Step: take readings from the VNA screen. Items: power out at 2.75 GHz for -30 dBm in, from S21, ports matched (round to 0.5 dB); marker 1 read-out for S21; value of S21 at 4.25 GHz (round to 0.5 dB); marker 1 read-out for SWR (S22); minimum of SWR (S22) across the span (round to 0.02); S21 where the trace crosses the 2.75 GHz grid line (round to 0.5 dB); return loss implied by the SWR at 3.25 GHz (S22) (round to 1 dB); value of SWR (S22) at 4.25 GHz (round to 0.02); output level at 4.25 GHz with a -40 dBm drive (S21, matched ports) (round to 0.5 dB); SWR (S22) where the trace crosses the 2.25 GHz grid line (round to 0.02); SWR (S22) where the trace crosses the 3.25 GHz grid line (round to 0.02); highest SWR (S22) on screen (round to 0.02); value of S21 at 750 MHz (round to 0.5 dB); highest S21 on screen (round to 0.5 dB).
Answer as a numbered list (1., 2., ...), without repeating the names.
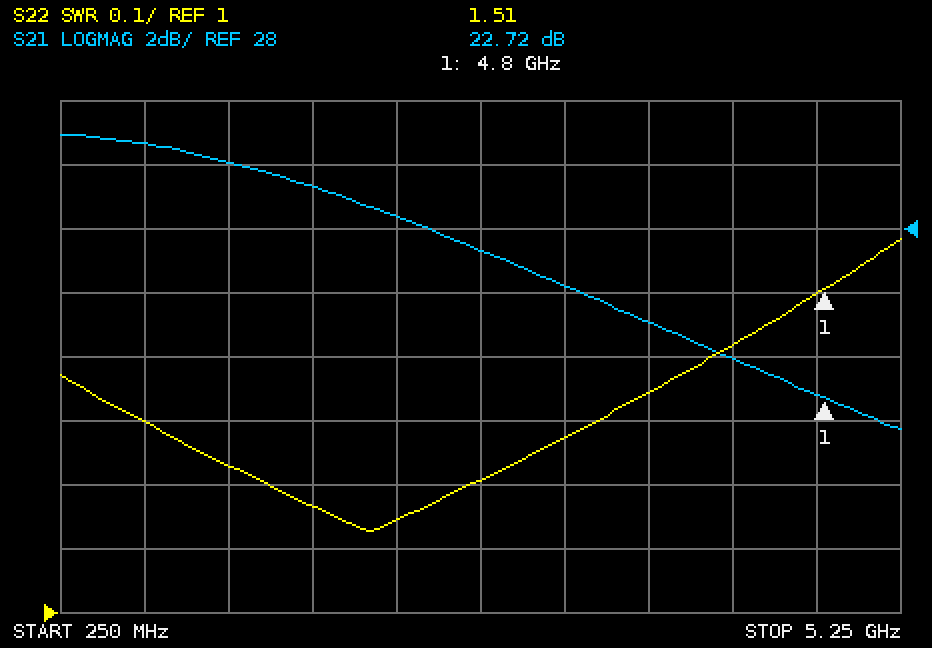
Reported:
1. -2.5 dBm
2. 22.72 dB
3. 24.0 dB
4. 1.51
5. 1.12
6. 27.5 dB
7. 18 dB
8. 1.42
9. -16.0 dBm
10. 1.14
11. 1.28
12. 1.58
13. 30.5 dB
14. 31.0 dB
